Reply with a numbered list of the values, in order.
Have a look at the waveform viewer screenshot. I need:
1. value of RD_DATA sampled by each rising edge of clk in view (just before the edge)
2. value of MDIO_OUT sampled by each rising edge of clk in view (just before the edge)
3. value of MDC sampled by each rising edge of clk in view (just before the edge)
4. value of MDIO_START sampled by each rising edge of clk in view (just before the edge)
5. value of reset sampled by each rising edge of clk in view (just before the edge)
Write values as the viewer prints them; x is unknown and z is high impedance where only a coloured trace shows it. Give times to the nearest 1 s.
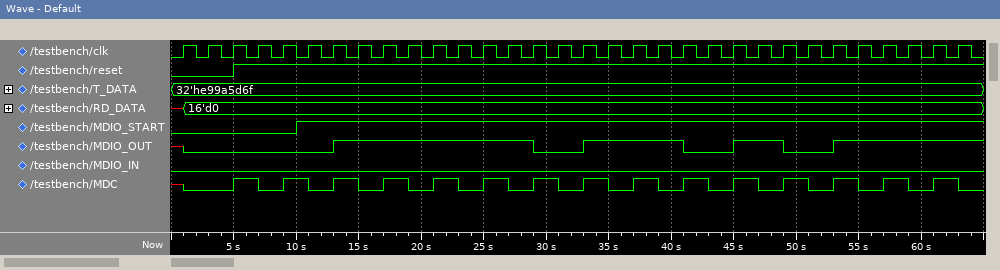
1. x, 16'd0, 16'd0, 16'd0, 16'd0, 16'd0, 16'd0, 16'd0, 16'd0, 16'd0, 16'd0, 16'd0, 16'd0, 16'd0, 16'd0, 16'd0, 16'd0, 16'd0, 16'd0, 16'd0, 16'd0, 16'd0, 16'd0, 16'd0, 16'd0, 16'd0, 16'd0, 16'd0, 16'd0, 16'd0, 16'd0, 16'd0
2. x 0 0 0 0 0 0 1 1 1 1 1 1 1 1 0 0 1 1 1 1 0 0 1 1 0 0 1 1 1 1 1
3. x 0 0 1 0 1 0 1 0 1 0 1 0 1 0 1 0 1 0 1 0 1 0 1 0 1 0 1 0 1 0 1
4. 0 0 0 0 0 1 1 1 1 1 1 1 1 1 1 1 1 1 1 1 1 1 1 1 1 1 1 1 1 1 1 1
5. 0 0 0 1 1 1 1 1 1 1 1 1 1 1 1 1 1 1 1 1 1 1 1 1 1 1 1 1 1 1 1 1
